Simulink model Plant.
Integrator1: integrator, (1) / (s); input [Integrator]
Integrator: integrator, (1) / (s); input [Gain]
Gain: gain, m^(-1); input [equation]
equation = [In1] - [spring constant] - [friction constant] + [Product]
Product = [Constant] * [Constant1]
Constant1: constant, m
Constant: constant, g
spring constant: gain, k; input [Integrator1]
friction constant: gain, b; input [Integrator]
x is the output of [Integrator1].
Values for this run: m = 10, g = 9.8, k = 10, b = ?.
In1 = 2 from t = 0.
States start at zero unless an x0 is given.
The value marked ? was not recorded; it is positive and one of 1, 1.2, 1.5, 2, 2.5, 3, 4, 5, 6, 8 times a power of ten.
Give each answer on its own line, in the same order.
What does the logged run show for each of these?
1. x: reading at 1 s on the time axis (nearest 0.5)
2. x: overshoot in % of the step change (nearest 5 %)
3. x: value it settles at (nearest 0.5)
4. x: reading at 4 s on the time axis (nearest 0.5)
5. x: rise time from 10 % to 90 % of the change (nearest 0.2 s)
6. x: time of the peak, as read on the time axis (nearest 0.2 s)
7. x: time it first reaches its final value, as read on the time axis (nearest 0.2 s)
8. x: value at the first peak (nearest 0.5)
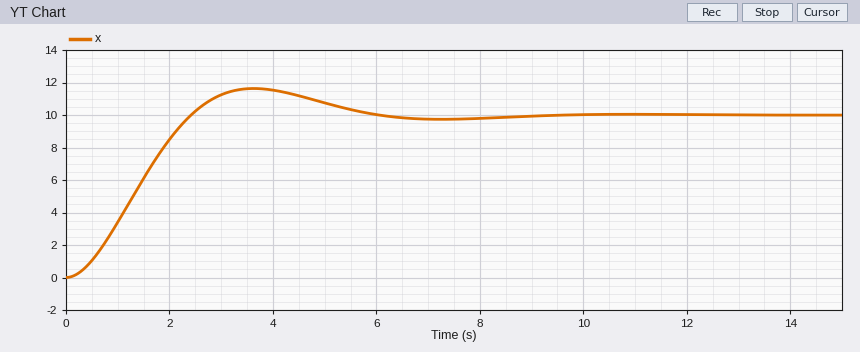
3.5
15 %
10.0
11.5
1.6 s
3.6 s
2.4 s
11.5
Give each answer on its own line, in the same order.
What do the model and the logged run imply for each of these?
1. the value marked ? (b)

10
